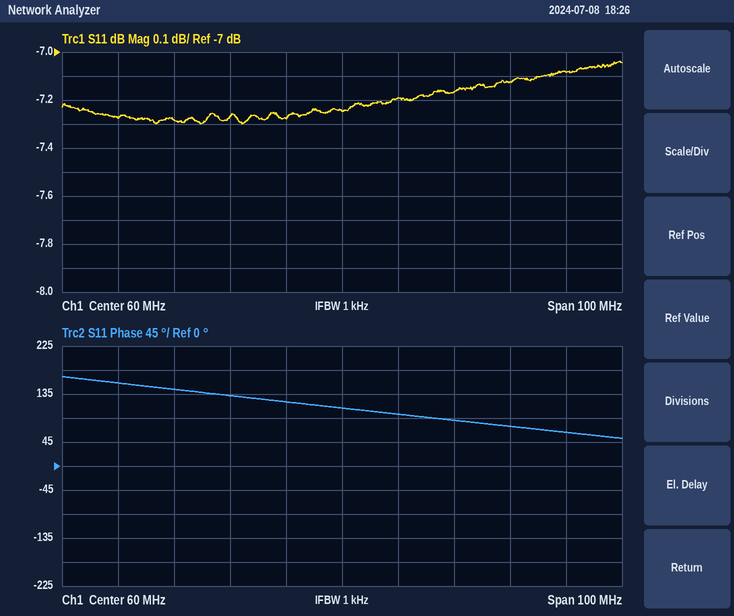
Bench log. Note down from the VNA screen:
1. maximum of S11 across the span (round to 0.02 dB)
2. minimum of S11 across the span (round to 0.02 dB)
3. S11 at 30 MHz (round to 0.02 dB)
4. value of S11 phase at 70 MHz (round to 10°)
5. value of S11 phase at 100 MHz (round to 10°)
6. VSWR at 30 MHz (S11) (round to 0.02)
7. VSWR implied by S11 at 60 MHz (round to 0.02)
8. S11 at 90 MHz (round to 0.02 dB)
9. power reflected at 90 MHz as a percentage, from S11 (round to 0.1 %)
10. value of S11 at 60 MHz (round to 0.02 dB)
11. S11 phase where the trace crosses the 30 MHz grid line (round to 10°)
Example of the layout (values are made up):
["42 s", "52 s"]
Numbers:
["-7.04 dB", "-7.30 dB", "-7.28 dB", "100°", "60°", "2.52", "2.54", "-7.12 dB", "19.4 %", "-7.24 dB", "140°"]
